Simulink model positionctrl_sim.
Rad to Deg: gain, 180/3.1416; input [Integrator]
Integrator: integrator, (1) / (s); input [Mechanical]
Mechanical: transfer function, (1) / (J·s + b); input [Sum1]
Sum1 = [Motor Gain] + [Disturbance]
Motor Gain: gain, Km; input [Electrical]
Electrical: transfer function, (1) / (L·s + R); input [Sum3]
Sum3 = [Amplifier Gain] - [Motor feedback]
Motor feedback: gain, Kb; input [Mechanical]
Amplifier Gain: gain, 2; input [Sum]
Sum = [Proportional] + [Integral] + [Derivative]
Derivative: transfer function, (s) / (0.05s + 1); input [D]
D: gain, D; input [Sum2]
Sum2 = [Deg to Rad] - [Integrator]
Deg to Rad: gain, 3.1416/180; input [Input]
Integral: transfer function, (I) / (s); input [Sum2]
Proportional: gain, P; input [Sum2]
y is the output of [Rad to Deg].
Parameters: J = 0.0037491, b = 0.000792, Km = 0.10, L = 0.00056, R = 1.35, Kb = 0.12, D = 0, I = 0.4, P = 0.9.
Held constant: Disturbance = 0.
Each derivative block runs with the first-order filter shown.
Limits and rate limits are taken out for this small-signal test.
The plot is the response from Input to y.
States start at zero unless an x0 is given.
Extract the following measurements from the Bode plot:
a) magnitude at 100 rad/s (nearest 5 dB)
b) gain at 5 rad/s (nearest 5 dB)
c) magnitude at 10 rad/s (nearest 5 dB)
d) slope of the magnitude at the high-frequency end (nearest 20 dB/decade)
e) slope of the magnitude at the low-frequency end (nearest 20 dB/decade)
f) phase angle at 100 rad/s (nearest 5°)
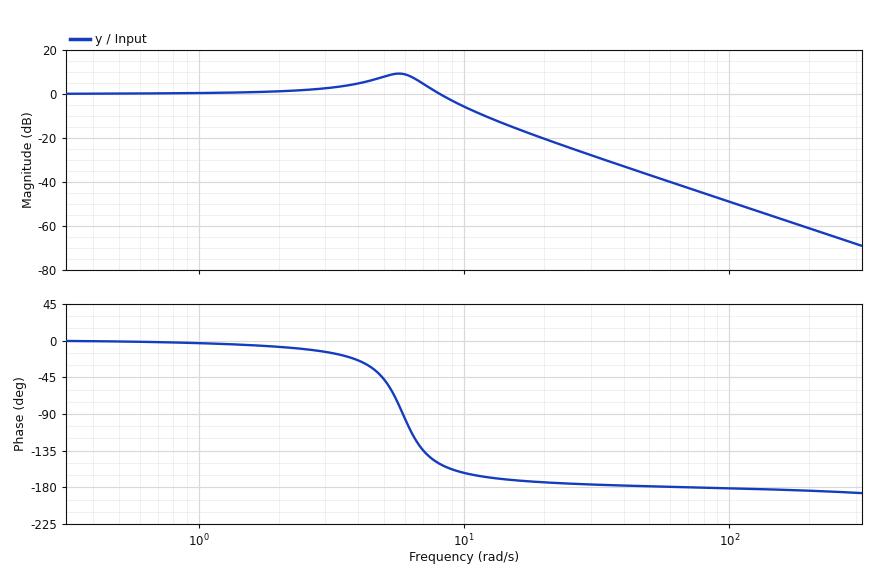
-50 dB
10 dB
-5 dB
-40 dB/decade
0 dB/decade
-180°
